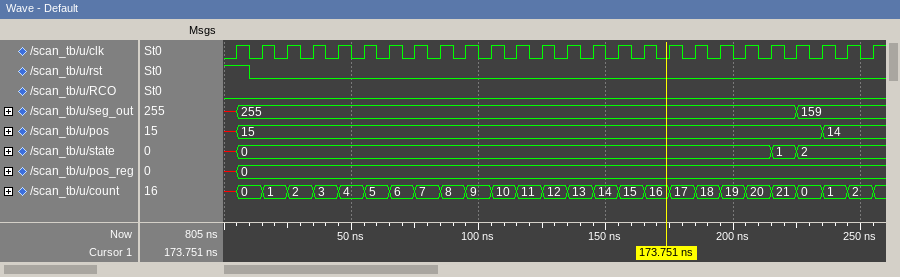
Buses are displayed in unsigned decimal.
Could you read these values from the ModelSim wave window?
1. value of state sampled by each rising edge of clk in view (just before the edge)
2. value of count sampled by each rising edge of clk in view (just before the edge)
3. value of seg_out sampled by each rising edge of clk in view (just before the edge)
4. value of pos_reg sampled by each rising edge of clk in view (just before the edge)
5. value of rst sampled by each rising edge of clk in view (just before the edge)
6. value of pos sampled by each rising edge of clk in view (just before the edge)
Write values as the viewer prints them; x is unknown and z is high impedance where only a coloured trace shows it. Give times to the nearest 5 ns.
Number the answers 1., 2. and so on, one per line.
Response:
1. x, 0, 0, 0, 0, 0, 0, 0, 0, 0, 0, 0, 0, 0, 0, 0, 0, 0, 0, 0, 0, 0, 1, 2, 2, 2
2. x, 0, 1, 2, 3, 4, 5, 6, 7, 8, 9, 10, 11, 12, 13, 14, 15, 16, 17, 18, 19, 20, 21, 0, 1, 2
3. x, 255, 255, 255, 255, 255, 255, 255, 255, 255, 255, 255, 255, 255, 255, 255, 255, 255, 255, 255, 255, 255, 255, 159, 159, 159
4. x, 0, 0, 0, 0, 0, 0, 0, 0, 0, 0, 0, 0, 0, 0, 0, 0, 0, 0, 0, 0, 0, 0, 0, 0, 0
5. 1 0 0 0 0 0 0 0 0 0 0 0 0 0 0 0 0 0 0 0 0 0 0 0 0 0
6. x, 15, 15, 15, 15, 15, 15, 15, 15, 15, 15, 15, 15, 15, 15, 15, 15, 15, 15, 15, 15, 15, 15, 15, 14, 14
